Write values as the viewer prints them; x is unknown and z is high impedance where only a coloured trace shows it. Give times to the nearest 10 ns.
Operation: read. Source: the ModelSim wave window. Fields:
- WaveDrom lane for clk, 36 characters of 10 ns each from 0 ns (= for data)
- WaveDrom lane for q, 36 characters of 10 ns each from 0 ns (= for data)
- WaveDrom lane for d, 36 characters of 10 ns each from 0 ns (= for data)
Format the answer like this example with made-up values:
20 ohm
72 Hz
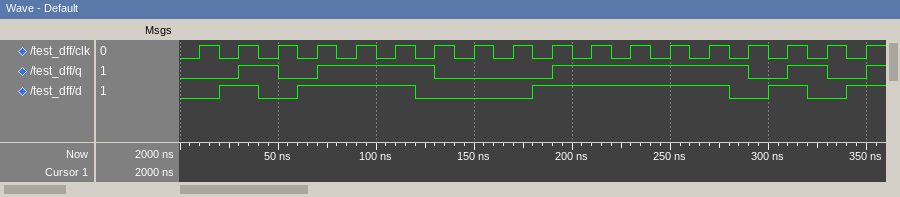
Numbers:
{name: 'clk', wave: '010101010101010101010101010101010101'}
{name: 'q', wave: '0..1.0.1.....0.....1.........0.1.0.1'}
{name: 'd', wave: '0.1.0.1.....0.....1.........0.1.0.1.'}
